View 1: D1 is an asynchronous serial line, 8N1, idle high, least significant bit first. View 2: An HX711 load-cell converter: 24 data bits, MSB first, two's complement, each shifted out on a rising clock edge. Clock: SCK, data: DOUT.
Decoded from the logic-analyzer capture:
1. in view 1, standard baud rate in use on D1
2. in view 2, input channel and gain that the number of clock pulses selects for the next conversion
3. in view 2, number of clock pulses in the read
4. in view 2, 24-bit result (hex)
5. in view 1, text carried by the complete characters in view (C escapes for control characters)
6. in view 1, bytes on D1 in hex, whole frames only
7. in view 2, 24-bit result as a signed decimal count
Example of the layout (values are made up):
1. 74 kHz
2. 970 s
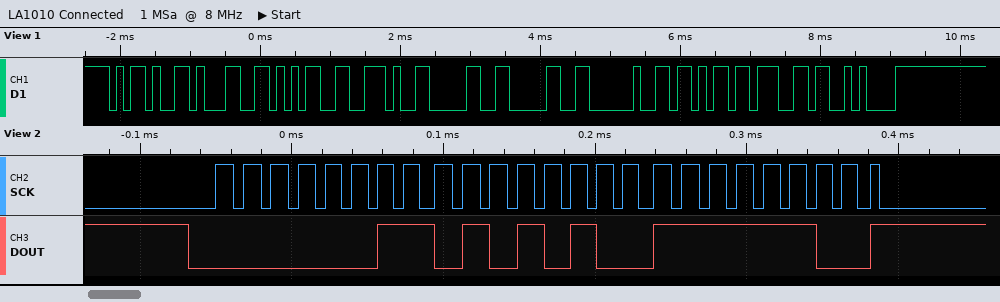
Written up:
1. 9600 baud
2. channel A, gain 128
3. 25
4. 0x0354FC
5. "-15.00 kg\n"
6. 2D 31 35 2E 30 30 20 6B 67 0A
7. 218364
